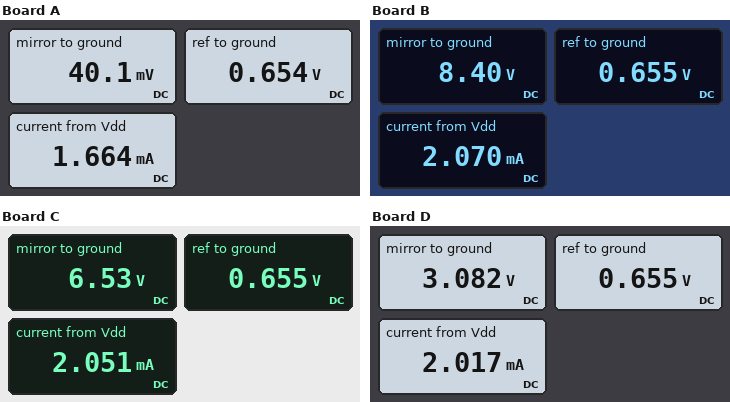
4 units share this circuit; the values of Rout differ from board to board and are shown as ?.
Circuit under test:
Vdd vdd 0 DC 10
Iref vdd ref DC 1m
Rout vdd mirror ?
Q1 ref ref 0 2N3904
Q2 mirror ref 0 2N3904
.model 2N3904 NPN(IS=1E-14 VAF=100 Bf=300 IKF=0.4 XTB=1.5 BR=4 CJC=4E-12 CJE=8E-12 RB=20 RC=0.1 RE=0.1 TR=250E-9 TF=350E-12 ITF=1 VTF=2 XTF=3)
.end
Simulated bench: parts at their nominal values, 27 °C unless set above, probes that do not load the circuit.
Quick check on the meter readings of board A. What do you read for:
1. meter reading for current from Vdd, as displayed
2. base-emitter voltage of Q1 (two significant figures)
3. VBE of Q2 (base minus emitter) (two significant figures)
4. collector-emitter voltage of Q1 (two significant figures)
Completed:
1.664 mA
650 mV
650 mV
650 mV
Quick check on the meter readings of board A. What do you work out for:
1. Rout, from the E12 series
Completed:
15 kΩ
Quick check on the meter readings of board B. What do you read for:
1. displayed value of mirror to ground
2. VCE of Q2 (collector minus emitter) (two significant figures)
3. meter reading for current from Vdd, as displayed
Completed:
8.40 V
8.4 V
2.070 mA
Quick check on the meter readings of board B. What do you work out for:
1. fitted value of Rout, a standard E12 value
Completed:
1.5 kΩ
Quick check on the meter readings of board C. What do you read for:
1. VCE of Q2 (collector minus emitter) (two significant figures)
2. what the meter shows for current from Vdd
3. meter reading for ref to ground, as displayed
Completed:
6.5 V
2.051 mA
0.655 V
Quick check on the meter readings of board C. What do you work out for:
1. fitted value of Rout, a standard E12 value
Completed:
3.3 kΩ
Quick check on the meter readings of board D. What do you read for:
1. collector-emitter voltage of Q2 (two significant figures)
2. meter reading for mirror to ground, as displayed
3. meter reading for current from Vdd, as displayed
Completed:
3.1 V
3.082 V
2.017 mA
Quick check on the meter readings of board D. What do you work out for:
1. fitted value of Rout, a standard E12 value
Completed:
6.8 kΩ
